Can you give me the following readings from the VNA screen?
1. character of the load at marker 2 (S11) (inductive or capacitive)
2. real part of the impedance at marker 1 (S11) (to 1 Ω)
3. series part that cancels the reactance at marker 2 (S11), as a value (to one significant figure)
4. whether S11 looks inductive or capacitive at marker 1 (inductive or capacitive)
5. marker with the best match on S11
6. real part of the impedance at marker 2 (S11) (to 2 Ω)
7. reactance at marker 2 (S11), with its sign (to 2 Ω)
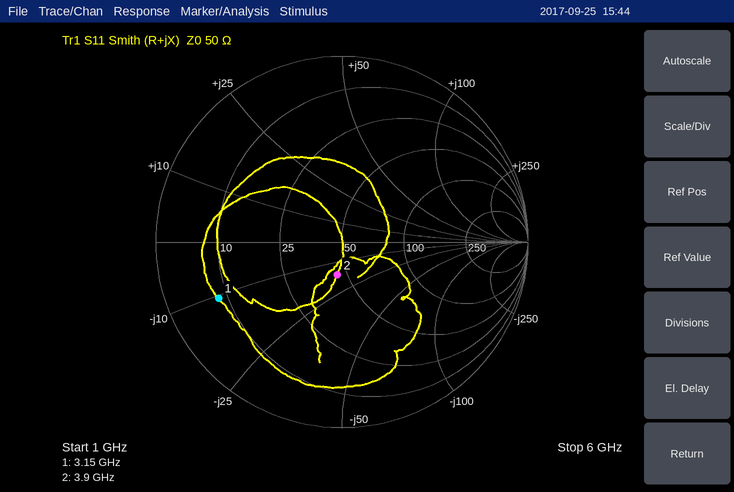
capacitive
8 Ω
700 pH
capacitive
marker 2
44 Ω
-16 Ω
